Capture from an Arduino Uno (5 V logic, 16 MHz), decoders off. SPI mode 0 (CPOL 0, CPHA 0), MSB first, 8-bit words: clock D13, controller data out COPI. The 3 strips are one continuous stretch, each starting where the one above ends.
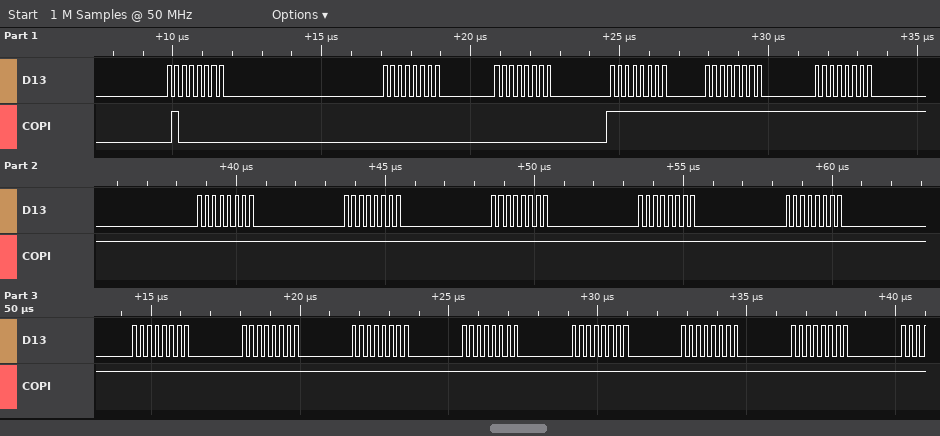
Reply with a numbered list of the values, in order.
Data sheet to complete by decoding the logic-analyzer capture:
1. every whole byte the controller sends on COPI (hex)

1. 40 00 00 FF FF FF FF FF FF FF FF FF FF FF FF FF FF FF
